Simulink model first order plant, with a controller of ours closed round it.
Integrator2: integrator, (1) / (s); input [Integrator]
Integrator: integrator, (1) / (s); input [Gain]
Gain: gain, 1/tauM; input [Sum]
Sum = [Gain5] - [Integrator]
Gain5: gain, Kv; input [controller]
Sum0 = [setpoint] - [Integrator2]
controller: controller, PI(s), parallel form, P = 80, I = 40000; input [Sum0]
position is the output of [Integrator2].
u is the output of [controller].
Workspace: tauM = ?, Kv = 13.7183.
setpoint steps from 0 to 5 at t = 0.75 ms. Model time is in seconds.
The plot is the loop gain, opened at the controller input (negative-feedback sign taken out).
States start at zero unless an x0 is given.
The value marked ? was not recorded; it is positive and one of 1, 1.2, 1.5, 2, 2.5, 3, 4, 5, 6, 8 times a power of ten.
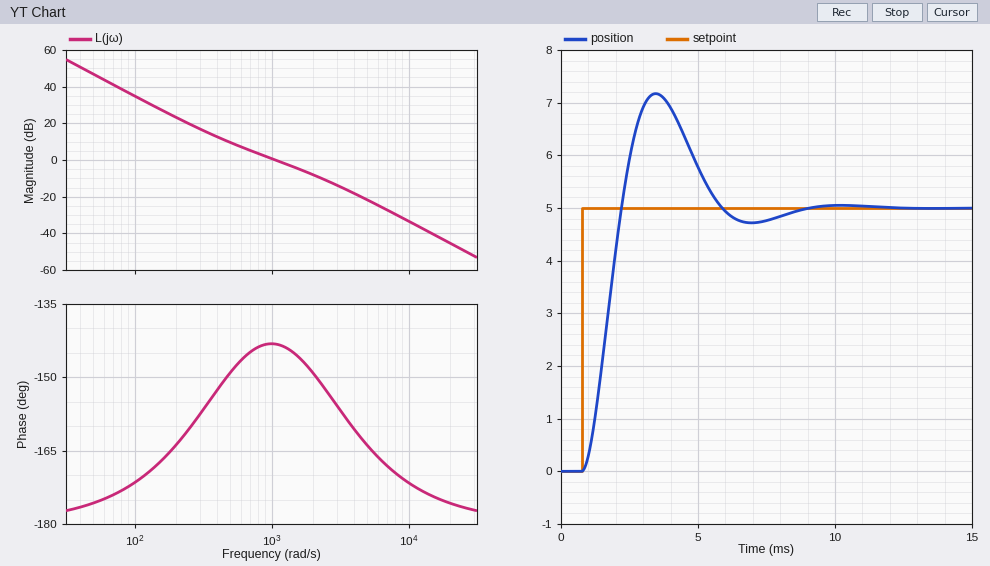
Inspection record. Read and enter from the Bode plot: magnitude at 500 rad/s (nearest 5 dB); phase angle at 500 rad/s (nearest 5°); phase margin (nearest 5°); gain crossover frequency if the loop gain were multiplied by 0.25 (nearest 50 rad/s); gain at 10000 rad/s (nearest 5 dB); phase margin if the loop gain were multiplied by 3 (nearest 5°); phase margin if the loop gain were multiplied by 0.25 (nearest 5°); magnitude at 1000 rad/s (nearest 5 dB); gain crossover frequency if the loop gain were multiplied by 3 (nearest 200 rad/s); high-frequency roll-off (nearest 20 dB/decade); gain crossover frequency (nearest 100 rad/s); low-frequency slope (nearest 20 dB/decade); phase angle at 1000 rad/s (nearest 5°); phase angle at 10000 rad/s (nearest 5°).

10 dB
-150°
35°
400 rad/s
-35 dB
30°
30°
0 dB
2200 rad/s
-40 dB/decade
1100 rad/s
-40 dB/decade
-145°
-170°
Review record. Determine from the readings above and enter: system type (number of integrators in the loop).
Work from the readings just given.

2
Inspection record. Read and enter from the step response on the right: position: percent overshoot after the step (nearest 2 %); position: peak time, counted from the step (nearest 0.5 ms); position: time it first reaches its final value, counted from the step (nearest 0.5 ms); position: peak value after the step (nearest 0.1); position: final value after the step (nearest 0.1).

44 %
2.5 ms
1.5 ms
7.2
5.0
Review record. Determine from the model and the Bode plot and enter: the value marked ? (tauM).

0.0005
